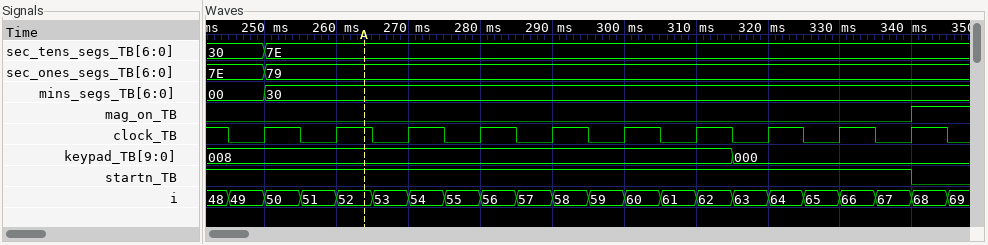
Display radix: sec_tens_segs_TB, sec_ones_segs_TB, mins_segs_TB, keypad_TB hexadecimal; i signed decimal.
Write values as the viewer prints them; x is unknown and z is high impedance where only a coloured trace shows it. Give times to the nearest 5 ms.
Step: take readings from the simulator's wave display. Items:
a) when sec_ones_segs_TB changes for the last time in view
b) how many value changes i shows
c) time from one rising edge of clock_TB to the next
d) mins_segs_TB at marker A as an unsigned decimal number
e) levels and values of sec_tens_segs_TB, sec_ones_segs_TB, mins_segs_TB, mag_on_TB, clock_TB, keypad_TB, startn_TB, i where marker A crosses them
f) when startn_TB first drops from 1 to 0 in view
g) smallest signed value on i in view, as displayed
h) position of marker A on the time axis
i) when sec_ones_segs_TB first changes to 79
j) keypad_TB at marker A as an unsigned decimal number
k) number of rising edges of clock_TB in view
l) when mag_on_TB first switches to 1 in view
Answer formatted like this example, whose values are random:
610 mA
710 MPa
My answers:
250 ms
21
10 ms
48
sec_tens_segs_TB=7E, sec_ones_segs_TB=79, mins_segs_TB=30, mag_on_TB=0, clock_TB=1, keypad_TB=008, startn_TB=1, i=52
340 ms
48
265 ms
250 ms
8
10
340 ms
